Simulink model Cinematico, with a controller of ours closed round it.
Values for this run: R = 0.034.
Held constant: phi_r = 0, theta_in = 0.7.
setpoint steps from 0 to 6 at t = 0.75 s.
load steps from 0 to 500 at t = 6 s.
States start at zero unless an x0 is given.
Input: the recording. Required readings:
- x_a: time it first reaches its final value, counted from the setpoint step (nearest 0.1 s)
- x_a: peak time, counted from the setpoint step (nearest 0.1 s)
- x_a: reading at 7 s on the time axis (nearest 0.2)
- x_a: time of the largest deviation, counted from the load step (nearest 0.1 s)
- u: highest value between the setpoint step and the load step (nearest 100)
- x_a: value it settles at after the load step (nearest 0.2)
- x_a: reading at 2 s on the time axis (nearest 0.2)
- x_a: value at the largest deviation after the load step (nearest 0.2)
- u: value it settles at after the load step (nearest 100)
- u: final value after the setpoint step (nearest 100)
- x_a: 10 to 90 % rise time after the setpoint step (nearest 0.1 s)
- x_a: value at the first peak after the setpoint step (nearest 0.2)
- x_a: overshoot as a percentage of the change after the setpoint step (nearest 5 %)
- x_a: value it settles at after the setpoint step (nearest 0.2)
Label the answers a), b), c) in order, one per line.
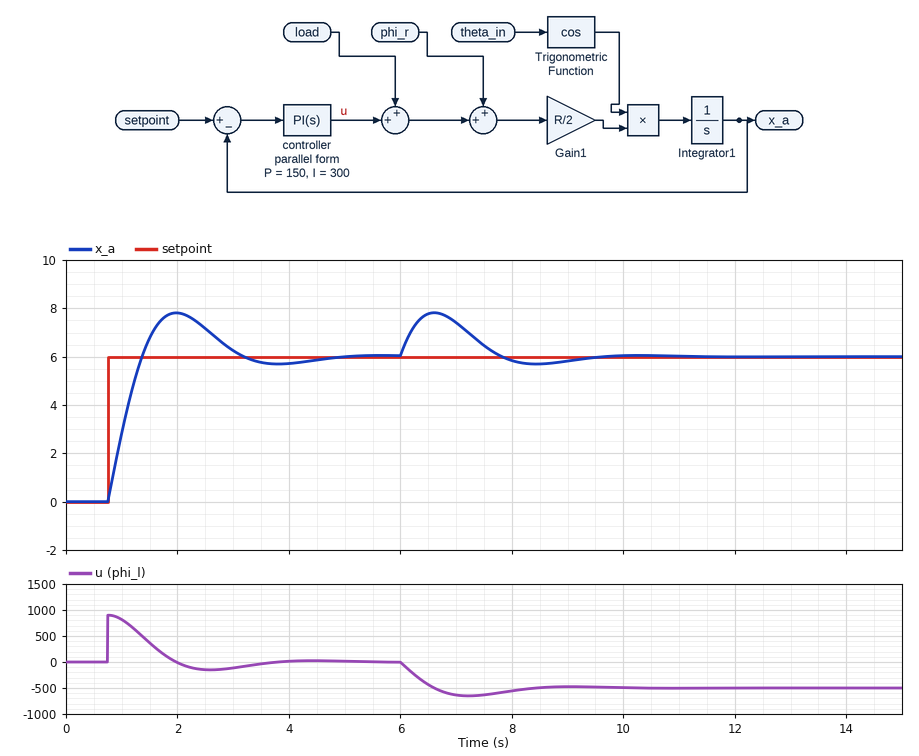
a) 0.6 s
b) 1.2 s
c) 7.4
d) 0.6 s
e) 900
f) 6.0
g) 7.8
h) 7.8
i) -500
j) 0
k) 0.5 s
l) 7.8
m) 30 %
n) 6.0
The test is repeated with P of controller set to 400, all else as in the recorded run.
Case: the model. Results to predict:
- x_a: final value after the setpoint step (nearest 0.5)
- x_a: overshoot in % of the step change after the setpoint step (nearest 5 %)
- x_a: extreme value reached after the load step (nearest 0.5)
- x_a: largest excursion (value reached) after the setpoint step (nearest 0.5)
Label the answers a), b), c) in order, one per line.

a) 6.0
b) 10 %
c) 7.0
d) 6.5
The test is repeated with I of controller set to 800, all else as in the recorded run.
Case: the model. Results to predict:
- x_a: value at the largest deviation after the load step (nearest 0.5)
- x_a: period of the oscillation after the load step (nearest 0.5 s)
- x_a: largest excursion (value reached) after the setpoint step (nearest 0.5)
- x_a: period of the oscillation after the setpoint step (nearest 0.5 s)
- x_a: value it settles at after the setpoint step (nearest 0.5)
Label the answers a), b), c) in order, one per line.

a) 7.5
b) 2.0 s
c) 8.5
d) 2.0 s
e) 6.0
